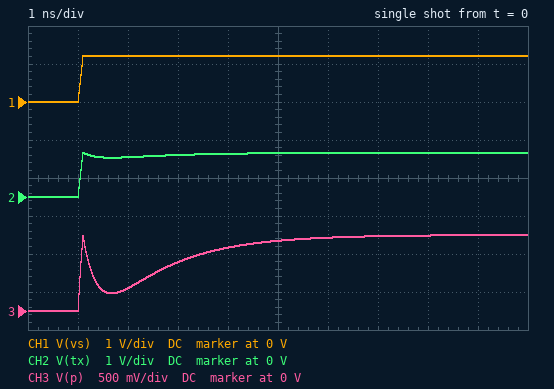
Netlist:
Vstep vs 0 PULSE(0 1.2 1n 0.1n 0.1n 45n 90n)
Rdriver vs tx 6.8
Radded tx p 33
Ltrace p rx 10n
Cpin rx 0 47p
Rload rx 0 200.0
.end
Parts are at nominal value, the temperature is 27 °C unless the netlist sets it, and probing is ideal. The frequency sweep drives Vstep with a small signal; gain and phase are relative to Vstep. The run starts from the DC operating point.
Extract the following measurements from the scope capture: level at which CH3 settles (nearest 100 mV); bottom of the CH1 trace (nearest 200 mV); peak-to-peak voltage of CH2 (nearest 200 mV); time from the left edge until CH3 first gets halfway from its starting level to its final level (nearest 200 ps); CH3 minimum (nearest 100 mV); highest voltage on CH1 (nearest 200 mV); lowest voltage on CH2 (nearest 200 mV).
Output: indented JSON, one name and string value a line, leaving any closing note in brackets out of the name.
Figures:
{
  "level at which CH3 settles": "1.0 V",
  "bottom of the CH1 trace": "0 V",
  "peak-to-peak voltage of CH2": "1.2 V",
  "time from the left edge until CH3 first gets halfway from its starting level to its final level": "1.0 ns",
  "CH3 minimum": "0 V",
  "highest voltage on CH1": "1.2 V",
  "lowest voltage on CH2": "0 V"
}
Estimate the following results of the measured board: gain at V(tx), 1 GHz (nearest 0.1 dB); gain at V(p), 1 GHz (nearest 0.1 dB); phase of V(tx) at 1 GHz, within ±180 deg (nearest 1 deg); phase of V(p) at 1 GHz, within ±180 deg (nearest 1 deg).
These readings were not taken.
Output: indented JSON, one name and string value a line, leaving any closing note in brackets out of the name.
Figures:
{
  "gain at V(tx), 1 GHz": "-0.4 dB",
  "gain at V(p), 1 GHz": "-1.6 dB",
  "phase of V(tx) at 1 GHz, within ±180 deg": "5 deg",
  "phase of V(p) at 1 GHz, within ±180 deg": "34 deg"
}
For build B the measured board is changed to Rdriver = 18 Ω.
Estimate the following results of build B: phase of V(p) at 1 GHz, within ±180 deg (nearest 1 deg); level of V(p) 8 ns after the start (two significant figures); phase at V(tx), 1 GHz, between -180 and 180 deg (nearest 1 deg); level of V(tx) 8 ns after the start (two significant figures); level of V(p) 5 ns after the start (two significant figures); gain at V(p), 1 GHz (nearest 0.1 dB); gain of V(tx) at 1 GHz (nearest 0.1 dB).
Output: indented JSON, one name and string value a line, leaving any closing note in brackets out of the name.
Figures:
{
  "phase of V(p) at 1 GHz, within ±180 deg": "41 deg",
  "level of V(p) 8 ns after the start": "930 mV",
  "phase at V(tx), 1 GHz, between -180 and 180 deg": "12 deg",
  "level of V(tx) 8 ns after the start": "1.1 V",
  "level of V(p) 5 ns after the start": "830 mV",
  "gain at V(p), 1 GHz": "-2.4 dB",
  "gain of V(tx) at 1 GHz": "-1.2 dB"
}
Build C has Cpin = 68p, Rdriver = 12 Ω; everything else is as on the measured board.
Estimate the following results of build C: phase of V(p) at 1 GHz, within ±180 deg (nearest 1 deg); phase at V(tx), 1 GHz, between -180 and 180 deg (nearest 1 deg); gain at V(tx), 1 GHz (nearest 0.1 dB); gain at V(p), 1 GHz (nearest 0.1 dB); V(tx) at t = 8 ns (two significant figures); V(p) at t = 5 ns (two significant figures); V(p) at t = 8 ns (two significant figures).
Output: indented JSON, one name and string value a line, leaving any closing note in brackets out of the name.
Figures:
{
  "phase of V(p) at 1 GHz, within ±180 deg": "37 deg",
  "phase at V(tx), 1 GHz, between -180 and 180 deg": "8 deg",
  "gain at V(tx), 1 GHz": "-0.8 dB",
  "gain at V(p), 1 GHz": "-1.9 dB",
  "V(tx) at t = 8 ns": "1.1 V",
  "V(p) at t = 5 ns": "760 mV",
  "V(p) at t = 8 ns": "920 mV"
}
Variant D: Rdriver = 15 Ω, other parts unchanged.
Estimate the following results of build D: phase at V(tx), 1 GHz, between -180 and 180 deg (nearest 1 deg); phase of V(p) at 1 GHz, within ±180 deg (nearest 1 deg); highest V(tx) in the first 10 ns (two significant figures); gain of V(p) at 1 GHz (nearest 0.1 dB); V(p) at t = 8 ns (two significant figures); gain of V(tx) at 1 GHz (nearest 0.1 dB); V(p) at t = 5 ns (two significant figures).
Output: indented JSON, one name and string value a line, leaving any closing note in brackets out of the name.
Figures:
{
  "phase at V(tx), 1 GHz, between -180 and 180 deg": "10 deg",
  "phase of V(p) at 1 GHz, within ±180 deg": "39 deg",
  "highest V(tx) in the first 10 ns": "1.1 V",
  "gain of V(p) at 1 GHz": "-2.2 dB",
  "V(p) at t = 8 ns": "950 mV",
  "gain of V(tx) at 1 GHz": "-1.0 dB",
  "V(p) at t = 5 ns": "850 mV"
}
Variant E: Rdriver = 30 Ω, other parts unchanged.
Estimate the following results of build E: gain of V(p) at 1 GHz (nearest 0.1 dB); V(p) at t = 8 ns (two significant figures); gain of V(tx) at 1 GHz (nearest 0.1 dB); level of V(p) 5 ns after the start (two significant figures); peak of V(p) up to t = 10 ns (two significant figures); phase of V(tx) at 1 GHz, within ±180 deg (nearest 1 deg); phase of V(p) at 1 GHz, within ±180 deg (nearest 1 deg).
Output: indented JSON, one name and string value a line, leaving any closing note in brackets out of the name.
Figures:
{
  "gain of V(p) at 1 GHz": "-3.3 dB",
  "V(p) at t = 8 ns": "870 mV",
  "gain of V(tx) at 1 GHz": "-2.1 dB",
  "level of V(p) 5 ns after the start": "750 mV",
  "peak of V(p) up to t = 10 ns": "900 mV",
  "phase of V(tx) at 1 GHz, within ±180 deg": "18 deg",
  "phase of V(p) at 1 GHz, within ±180 deg": "47 deg"
}
